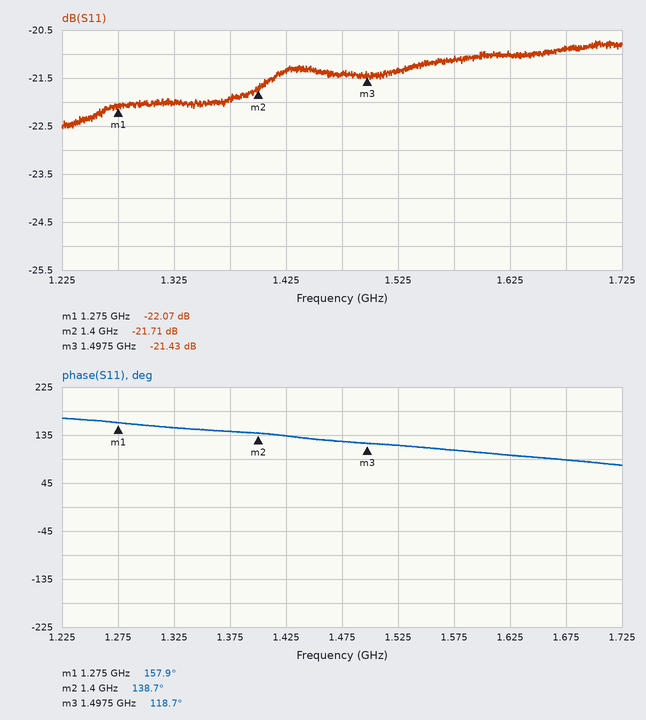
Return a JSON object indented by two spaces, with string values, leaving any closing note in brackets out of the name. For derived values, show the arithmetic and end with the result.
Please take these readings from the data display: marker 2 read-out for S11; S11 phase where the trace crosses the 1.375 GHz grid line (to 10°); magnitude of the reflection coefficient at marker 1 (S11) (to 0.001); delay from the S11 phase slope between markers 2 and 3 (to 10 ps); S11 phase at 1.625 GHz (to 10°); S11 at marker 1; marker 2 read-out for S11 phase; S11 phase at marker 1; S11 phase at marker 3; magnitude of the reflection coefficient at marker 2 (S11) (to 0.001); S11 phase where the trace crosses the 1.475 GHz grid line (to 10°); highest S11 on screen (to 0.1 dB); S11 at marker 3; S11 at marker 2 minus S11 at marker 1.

{
  "marker 2 read-out for S11": "-21.71 dB",
  "S11 phase where the trace crosses the 1.375 GHz grid line": "140°",
  "magnitude of the reflection coefficient at marker 1 (S11)": "10^(-22.07/20) ≈ 0.079",
  "delay from the S11 phase slope between markers 2 and 3": "−(118.7° − (138.7°))/(360° × 97.5 MHz) ≈ 570 ps",
  "S11 phase at 1.625 GHz": "100°",
  "S11 at marker 1": "-22.07 dB",
  "marker 2 read-out for S11 phase": "138.7°",
  "S11 phase at marker 1": "157.9°",
  "S11 phase at marker 3": "118.7°",
  "magnitude of the reflection coefficient at marker 2 (S11)": "10^(-21.71/20) ≈ 0.082",
  "S11 phase where the trace crosses the 1.475 GHz grid line": "120°",
  "highest S11 on screen": "-20.7 dB",
  "S11 at marker 3": "-21.43 dB",
  "S11 at marker 2 minus S11 at marker 1": "-21.71 − (-22.07) = 0.36 dB"
}
